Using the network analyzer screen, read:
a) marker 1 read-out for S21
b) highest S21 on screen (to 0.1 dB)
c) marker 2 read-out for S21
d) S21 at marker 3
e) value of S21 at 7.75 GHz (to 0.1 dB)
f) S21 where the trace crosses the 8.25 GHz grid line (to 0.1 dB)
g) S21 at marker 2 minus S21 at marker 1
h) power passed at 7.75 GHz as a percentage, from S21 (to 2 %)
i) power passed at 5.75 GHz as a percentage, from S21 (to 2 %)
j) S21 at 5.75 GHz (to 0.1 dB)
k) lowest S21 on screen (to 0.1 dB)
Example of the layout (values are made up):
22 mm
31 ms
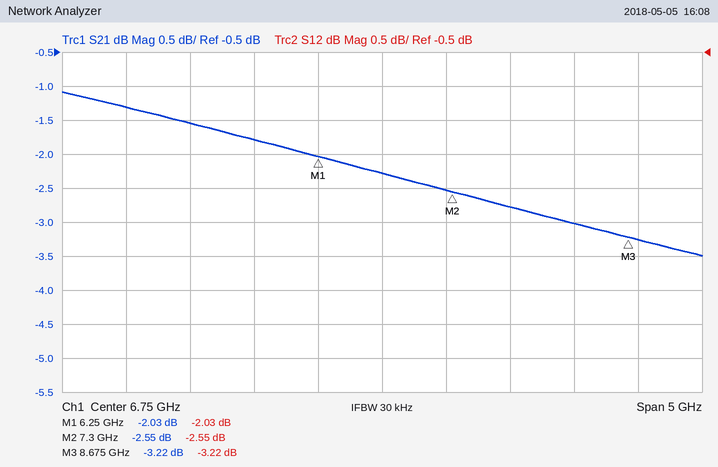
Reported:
-2.03 dB
-1.1 dB
-2.55 dB
-3.22 dB
-2.8 dB
-3.0 dB
-0.52 dB
52 %
66 %
-1.8 dB
-3.5 dB
